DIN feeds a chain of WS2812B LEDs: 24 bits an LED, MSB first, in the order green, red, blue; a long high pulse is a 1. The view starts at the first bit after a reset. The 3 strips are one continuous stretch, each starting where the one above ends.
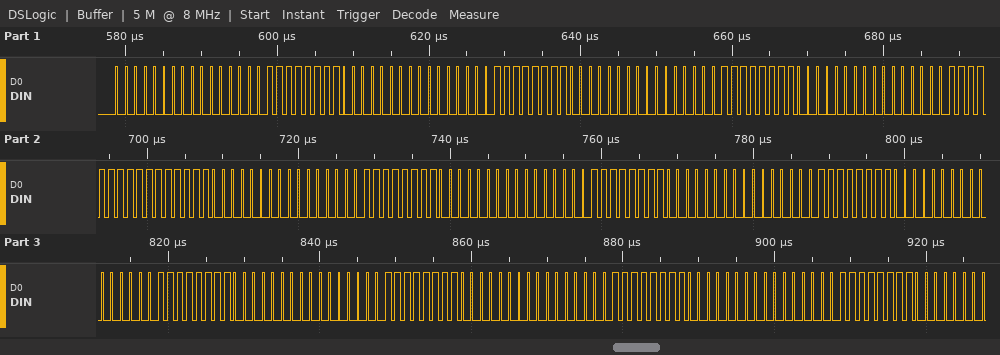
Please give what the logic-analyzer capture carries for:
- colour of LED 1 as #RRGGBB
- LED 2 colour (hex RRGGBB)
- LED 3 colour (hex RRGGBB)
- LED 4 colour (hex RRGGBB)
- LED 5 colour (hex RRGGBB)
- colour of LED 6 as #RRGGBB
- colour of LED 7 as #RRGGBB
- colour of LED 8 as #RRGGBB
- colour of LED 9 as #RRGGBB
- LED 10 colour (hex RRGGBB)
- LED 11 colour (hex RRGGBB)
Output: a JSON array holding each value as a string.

["#0000FF", "#0000FF", "#0000FF", "#0000FF", "#00FF00", "#00FF00", "#00FF00", "#00FF00", "#00FF00", "#00FF00", "#00FF00"]
